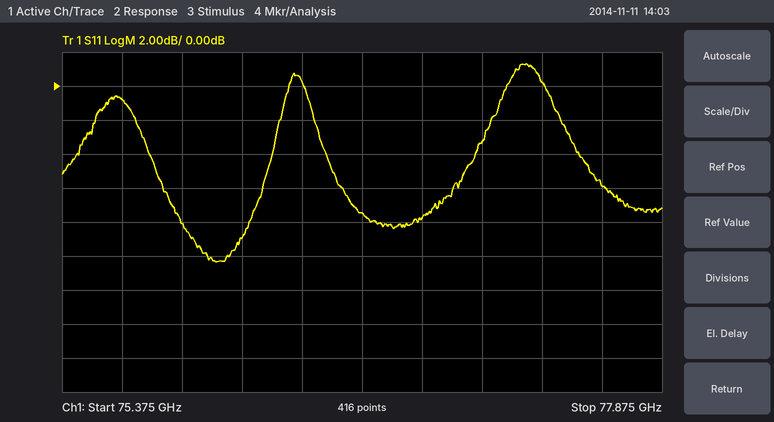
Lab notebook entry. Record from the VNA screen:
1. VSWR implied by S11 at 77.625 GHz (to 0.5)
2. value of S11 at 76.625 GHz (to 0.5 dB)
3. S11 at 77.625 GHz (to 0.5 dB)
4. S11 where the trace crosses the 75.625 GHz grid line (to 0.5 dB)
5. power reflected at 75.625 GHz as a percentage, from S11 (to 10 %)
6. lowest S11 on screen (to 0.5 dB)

3.0
-7.5 dB
-6.0 dB
-1.0 dB
80 %
-10.5 dB
